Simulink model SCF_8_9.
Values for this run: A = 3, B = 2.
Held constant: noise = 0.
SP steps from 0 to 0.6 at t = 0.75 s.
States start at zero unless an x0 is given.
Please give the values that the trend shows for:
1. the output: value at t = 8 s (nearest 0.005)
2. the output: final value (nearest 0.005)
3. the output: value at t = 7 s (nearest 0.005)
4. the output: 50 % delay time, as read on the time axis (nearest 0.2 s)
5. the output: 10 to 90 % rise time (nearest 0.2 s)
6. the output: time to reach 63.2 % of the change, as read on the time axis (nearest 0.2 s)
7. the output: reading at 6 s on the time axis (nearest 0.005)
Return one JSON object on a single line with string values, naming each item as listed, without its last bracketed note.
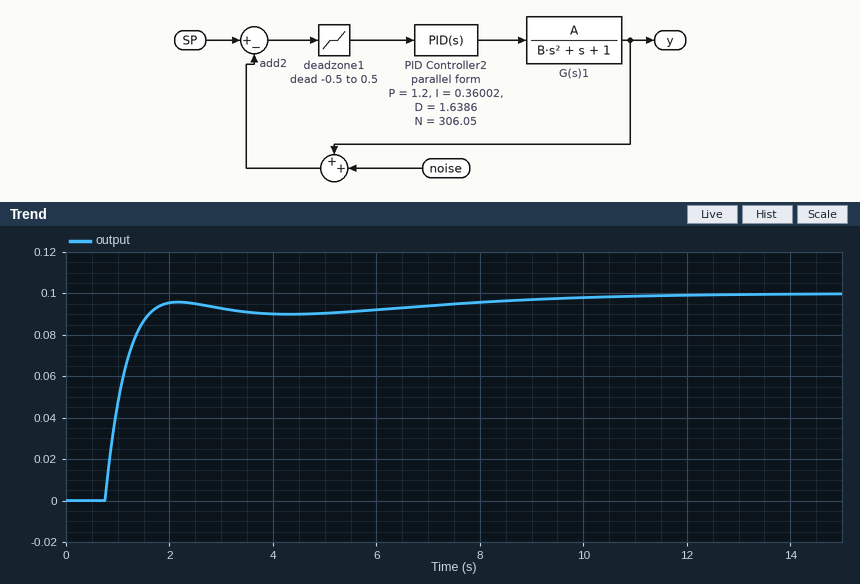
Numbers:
{"the output: value at t = 8 s": "0.095", "the output: final value": "0.100", "the output: value at t = 7 s": "0.095", "the output: 50 % delay time, as read on the time axis": "1.0 s", "the output: 10 to 90 % rise time": "0.8 s", "the output: time to reach 63.2 % of the change, as read on the time axis": "1.2 s", "the output: reading at 6 s on the time axis": "0.090"}
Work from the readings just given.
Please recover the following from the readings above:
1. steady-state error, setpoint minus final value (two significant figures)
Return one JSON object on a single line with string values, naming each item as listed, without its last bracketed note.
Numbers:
{"steady-state error, setpoint minus final value": "0.50"}
